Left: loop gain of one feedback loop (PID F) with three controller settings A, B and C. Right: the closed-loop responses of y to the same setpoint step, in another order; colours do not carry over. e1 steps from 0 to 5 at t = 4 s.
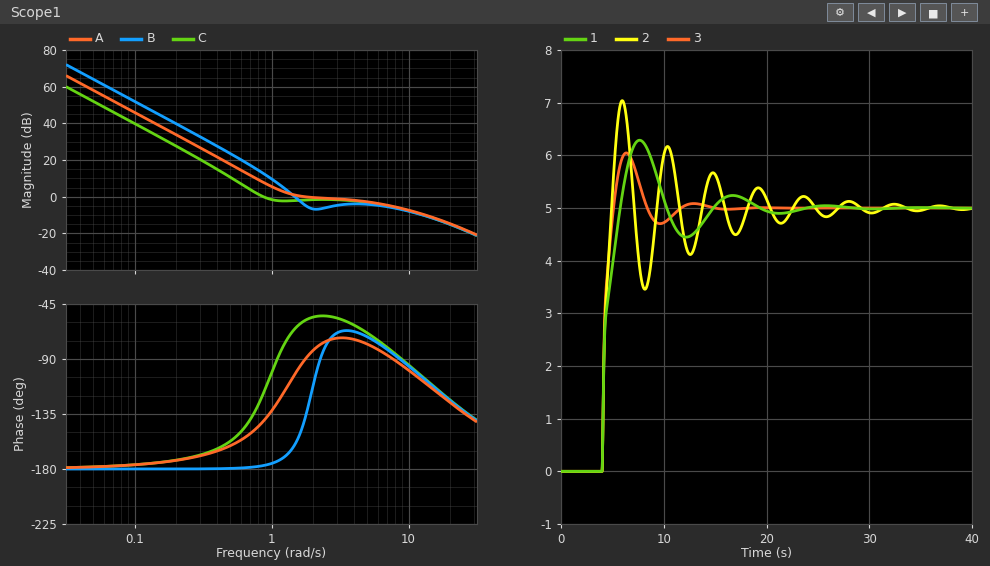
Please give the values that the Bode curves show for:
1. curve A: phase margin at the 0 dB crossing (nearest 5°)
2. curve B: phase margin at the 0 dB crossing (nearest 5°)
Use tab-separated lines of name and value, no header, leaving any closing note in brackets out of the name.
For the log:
curve A: phase margin at the 0 dB crossing	90°
curve B: phase margin at the 0 dB crossing	20°
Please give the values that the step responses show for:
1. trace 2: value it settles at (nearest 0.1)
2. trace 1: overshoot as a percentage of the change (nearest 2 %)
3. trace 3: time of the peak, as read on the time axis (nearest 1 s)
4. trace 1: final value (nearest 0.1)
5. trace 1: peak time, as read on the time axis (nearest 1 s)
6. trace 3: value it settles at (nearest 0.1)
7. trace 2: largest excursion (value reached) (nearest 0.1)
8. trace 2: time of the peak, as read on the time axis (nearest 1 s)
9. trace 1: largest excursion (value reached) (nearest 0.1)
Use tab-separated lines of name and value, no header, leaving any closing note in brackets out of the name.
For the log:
trace 2: value it settles at	5.0
trace 1: overshoot as a percentage of the change	26 %
trace 3: time of the peak, as read on the time axis	6 s
trace 1: final value	5.0
trace 1: peak time, as read on the time axis	8 s
trace 3: value it settles at	5.0
trace 2: largest excursion (value reached)	7.0
trace 2: time of the peak, as read on the time axis	6 s
trace 1: largest excursion (value reached)	6.3
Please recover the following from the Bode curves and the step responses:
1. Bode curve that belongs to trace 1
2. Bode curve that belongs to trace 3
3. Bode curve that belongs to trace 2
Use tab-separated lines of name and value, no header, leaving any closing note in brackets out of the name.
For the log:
Bode curve that belongs to trace 1	C
Bode curve that belongs to trace 3	A
Bode curve that belongs to trace 2	B
